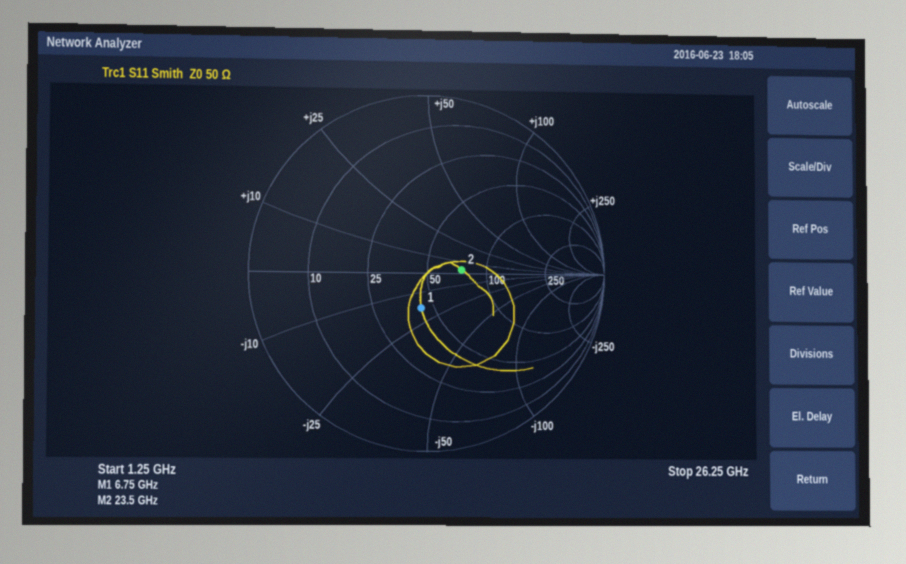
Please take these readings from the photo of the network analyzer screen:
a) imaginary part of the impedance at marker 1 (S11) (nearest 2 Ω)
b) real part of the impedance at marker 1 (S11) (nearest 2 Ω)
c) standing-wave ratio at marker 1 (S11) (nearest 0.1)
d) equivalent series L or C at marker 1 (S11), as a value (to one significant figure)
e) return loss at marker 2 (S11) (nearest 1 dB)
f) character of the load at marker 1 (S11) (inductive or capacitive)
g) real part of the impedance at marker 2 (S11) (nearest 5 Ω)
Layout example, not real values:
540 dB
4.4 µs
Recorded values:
-18 Ω
44 Ω
1.5
1 pF
14 dB
capacitive
75 Ω
